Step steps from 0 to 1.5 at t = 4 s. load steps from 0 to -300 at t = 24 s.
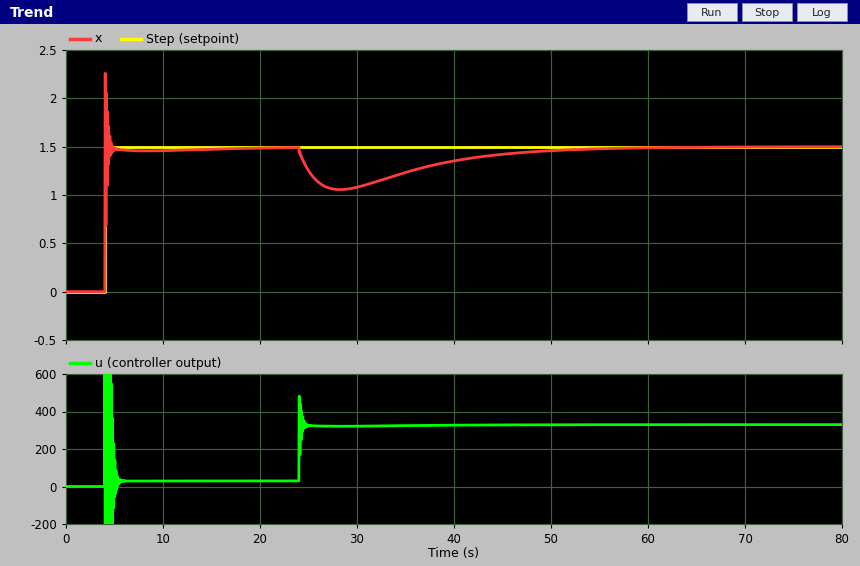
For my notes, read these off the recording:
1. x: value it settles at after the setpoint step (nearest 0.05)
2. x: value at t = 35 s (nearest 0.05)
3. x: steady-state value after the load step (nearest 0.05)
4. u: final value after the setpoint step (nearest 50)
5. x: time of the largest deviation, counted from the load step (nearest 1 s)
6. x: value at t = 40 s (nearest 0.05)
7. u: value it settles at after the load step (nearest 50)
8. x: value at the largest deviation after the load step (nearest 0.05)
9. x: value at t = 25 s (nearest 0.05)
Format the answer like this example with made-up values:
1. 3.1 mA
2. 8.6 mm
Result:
1. 1.50
2. 1.25
3. 1.50
4. 50
5. 4 s
6. 1.35
7. 350
8. 1.05
9. 1.25
